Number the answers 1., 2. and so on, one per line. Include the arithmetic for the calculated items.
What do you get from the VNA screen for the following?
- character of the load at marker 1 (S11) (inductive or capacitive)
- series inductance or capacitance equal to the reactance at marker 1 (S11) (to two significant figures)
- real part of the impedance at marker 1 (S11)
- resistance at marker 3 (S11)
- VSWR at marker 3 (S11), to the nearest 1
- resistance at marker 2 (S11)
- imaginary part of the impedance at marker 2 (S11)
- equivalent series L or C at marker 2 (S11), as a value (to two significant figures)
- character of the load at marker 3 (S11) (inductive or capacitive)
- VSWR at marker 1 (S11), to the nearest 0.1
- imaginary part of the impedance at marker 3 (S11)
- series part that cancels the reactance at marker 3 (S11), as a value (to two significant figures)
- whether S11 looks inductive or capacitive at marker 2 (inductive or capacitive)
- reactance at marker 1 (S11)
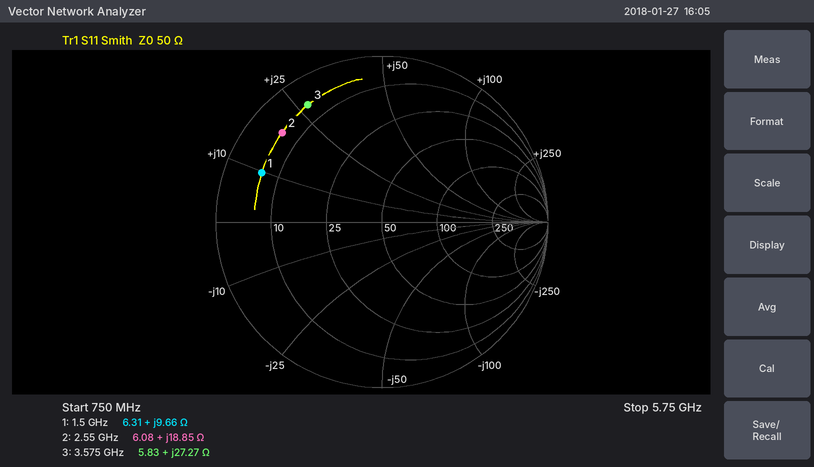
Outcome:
1. inductive
2. L = 9.66 Ω/(2π × 1.5 GHz) ≈ 1.0 nH
3. 6.31 Ω
4. 5.83 Ω
5. 11
6. 6.08 Ω
7. +18.85 Ω
8. L = 18.85 Ω/(2π × 2.55 GHz) ≈ 1.2 nH
9. inductive
10. 8.2
11. +27.27 Ω
12. C = 1/(2π × 3.575 GHz × 27.27 Ω) ≈ 1.6 pF
13. inductive
14. +9.66 Ω
